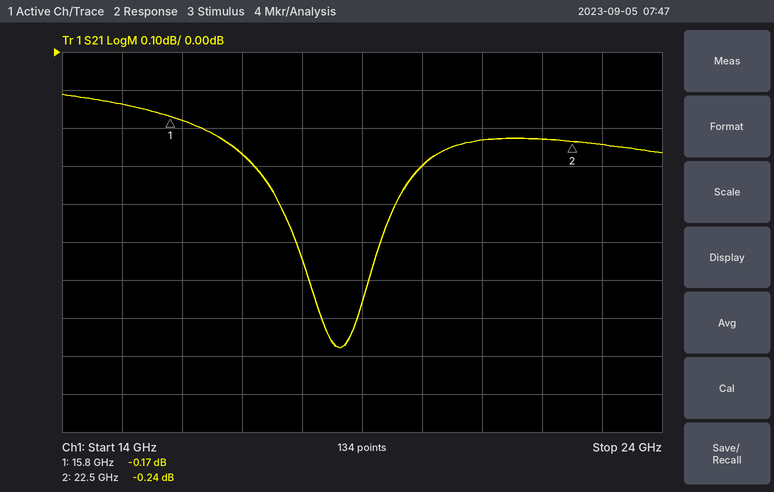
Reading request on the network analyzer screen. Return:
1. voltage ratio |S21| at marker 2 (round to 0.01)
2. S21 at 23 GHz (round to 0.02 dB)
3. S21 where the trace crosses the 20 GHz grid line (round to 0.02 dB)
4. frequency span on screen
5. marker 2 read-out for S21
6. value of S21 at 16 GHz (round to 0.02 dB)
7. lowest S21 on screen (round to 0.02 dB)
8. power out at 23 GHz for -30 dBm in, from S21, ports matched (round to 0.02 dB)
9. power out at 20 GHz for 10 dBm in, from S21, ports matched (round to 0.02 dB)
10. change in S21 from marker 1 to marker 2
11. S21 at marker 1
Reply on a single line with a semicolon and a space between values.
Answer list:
0.97; -0.24 dB; -0.30 dB; 10 GHz; -0.24 dB; -0.18 dB; -0.78 dB; -30.24 dBm; 9.70 dBm; -0.07 dB; -0.17 dB
